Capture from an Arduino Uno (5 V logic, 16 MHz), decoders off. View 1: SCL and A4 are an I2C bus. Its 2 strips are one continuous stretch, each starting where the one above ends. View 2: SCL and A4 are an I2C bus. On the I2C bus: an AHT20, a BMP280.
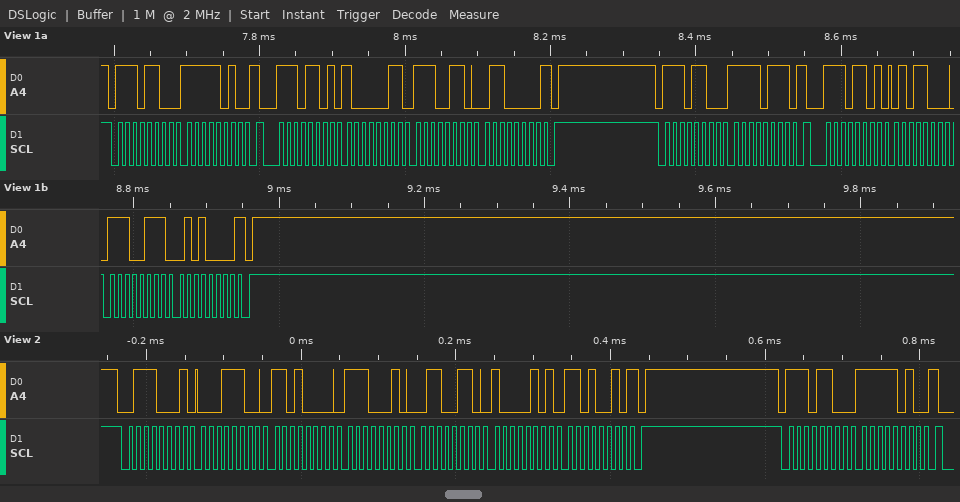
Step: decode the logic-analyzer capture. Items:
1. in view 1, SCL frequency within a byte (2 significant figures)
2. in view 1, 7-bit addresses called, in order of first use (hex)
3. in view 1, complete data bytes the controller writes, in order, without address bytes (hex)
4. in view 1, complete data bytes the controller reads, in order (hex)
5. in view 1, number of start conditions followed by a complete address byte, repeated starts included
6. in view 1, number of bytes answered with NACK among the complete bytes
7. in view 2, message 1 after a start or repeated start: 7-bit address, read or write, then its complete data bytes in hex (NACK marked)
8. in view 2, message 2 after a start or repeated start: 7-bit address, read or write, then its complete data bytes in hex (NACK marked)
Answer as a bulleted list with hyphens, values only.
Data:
- 100 kHz
- 0x76
- FA F7
- 83 E6 60 58 E7 50
- 4
- 2
- 0x38 read: 1C D0 E2 66 85 D2 NACK
- 0x76 write: FA
